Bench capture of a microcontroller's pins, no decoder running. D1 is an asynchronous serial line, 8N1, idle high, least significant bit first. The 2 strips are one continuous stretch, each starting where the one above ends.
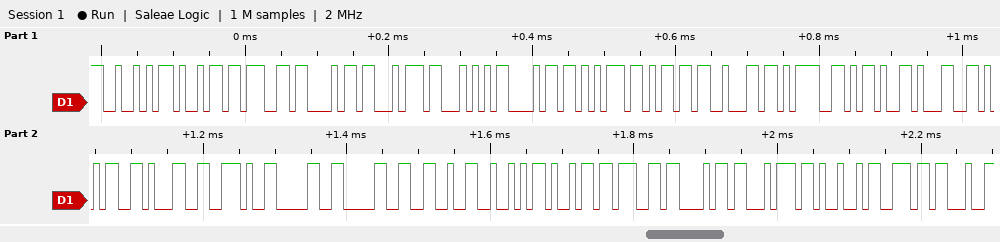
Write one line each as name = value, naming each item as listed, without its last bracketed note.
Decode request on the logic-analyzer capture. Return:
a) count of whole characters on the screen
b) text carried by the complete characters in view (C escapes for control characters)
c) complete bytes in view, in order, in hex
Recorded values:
count of whole characters on the screen = 26
text carried by the complete characters in view = "RightThumb=-151.00&RightIn"
complete bytes in view, in order, in hex = 0x52 0x69 0x67 0x68 0x74 0x54 0x68 0x75 0x6D 0x62 0x3D 0x2D 0x31 0x35 0x31 0x2E 0x30 0x30 0x26 0x52 0x69 0x67 0x68 0x74 0x49 0x6E
